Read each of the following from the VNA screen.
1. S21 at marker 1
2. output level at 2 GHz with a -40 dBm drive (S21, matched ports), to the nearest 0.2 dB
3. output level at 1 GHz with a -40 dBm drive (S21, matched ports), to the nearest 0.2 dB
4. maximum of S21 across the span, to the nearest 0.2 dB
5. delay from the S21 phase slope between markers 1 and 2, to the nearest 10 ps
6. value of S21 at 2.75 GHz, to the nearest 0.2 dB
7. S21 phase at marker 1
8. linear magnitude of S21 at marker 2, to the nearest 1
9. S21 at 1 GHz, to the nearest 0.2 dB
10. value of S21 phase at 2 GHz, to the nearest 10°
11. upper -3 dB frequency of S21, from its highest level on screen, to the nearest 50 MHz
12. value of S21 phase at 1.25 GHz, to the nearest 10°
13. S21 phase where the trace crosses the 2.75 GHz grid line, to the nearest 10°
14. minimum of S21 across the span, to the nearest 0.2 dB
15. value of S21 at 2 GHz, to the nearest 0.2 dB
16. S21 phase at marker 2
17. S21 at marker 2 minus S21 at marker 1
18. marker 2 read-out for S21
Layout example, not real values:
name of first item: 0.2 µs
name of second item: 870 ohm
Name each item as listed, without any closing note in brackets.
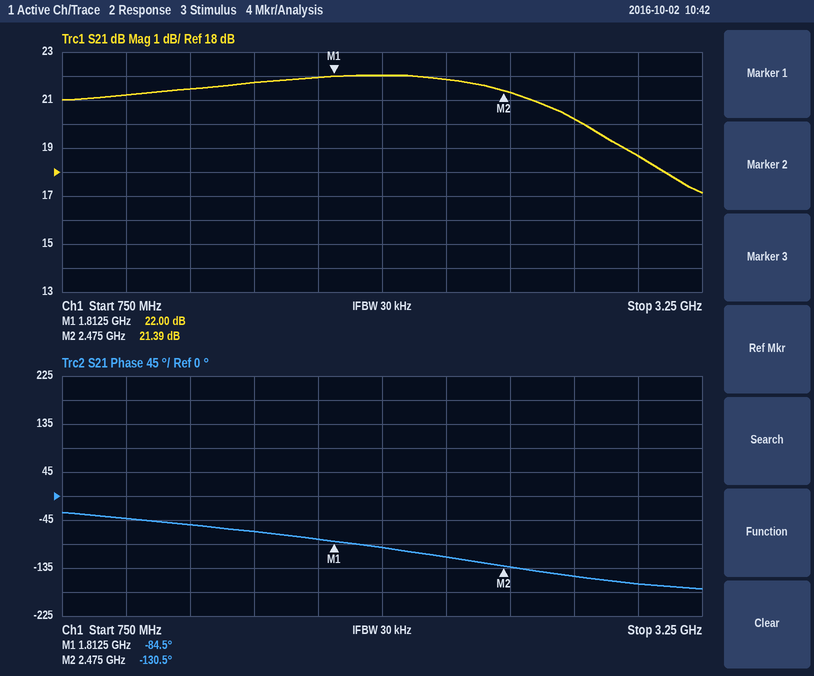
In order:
S21 at marker 1: 22.00 dB
output level at 2 GHz with a -40 dBm drive (S21, matched ports), to the nearest 0.2 dB: -18.0 dBm
output level at 1 GHz with a -40 dBm drive (S21, matched ports), to the nearest 0.2 dB: -18.8 dBm
maximum of S21 across the span, to the nearest 0.2 dB: 22.0 dB
delay from the S21 phase slope between markers 1 and 2, to the nearest 10 ps: 190 ps
value of S21 at 2.75 GHz, to the nearest 0.2 dB: 20.2 dB
S21 phase at marker 1: -84.5°
linear magnitude of S21 at marker 2, to the nearest 1: 12
S21 at 1 GHz, to the nearest 0.2 dB: 21.2 dB
value of S21 phase at 2 GHz, to the nearest 10°: -100°
upper -3 dB frequency of S21, from its highest level on screen, to the nearest 50 MHz: 2.95 GHz
value of S21 phase at 1.25 GHz, to the nearest 10°: -50°
S21 phase where the trace crosses the 2.75 GHz grid line, to the nearest 10°: -150°
minimum of S21 across the span, to the nearest 0.2 dB: 17.2 dB
value of S21 at 2 GHz, to the nearest 0.2 dB: 22.0 dB
S21 phase at marker 2: -130.5°
S21 at marker 2 minus S21 at marker 1: -0.61 dB
marker 2 read-out for S21: 21.39 dB
